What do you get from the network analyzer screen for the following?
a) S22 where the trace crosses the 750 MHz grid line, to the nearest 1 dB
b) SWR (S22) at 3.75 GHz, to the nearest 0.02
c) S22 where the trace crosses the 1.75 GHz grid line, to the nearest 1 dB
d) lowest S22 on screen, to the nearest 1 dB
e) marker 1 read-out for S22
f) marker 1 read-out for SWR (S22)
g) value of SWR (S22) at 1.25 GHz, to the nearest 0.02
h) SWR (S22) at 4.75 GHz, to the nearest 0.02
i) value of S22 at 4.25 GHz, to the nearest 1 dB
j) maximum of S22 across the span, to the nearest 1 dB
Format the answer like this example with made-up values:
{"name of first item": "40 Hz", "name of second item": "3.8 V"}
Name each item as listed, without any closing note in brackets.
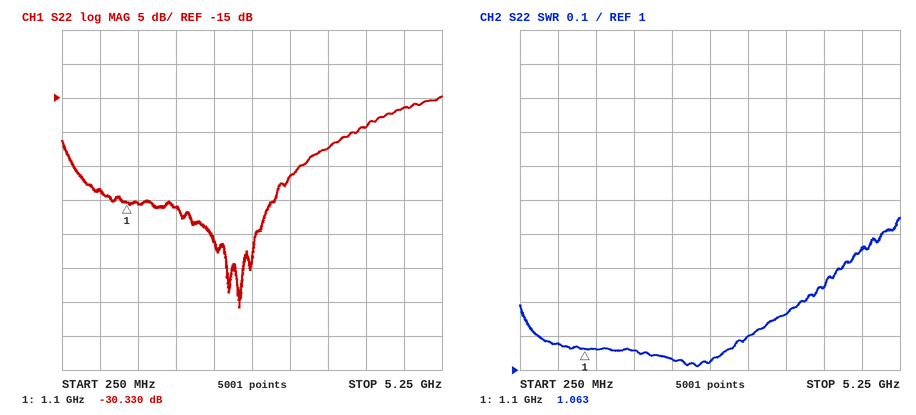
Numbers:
{"S22 where the trace crosses the 750 MHz grid line, to the nearest 1 dB": "-29 dB", "SWR (S22) at 3.75 GHz, to the nearest 0.02": "1.16", "S22 where the trace crosses the 1.75 GHz grid line, to the nearest 1 dB": "-31 dB", "lowest S22 on screen, to the nearest 1 dB": "-46 dB", "marker 1 read-out for S22": "-30.330 dB", "marker 1 read-out for SWR": "1.063", "value of SWR (S22) at 1.25 GHz, to the nearest 0.02": "1.06", "SWR (S22) at 4.75 GHz, to the nearest 0.02": "1.36", "value of S22 at 4.25 GHz, to the nearest 1 dB": "-19 dB", "maximum of S22 across the span, to the nearest 1 dB": "-15 dB"}
